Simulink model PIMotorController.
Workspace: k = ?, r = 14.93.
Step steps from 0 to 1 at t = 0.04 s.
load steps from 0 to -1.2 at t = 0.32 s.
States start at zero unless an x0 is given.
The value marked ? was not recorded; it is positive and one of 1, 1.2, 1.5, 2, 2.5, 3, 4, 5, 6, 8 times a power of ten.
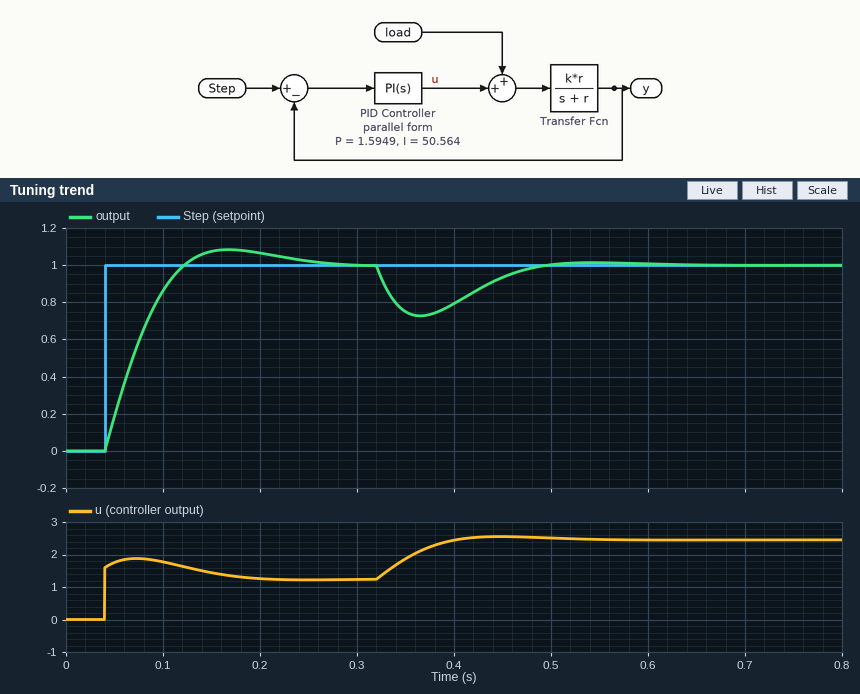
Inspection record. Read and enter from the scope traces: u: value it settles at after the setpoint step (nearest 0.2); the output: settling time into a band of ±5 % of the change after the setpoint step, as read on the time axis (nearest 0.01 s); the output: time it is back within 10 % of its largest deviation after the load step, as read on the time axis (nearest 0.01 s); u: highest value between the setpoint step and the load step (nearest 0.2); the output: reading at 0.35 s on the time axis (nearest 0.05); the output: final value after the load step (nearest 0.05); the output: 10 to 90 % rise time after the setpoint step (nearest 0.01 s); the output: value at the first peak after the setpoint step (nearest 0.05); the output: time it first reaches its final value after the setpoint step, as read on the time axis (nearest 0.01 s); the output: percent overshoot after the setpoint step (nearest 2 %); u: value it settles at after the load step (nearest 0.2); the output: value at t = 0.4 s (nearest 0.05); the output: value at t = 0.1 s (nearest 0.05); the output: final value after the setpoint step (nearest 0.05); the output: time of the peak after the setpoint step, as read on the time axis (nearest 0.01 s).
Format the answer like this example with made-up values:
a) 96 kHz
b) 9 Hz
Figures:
a) 1.2
b) 0.22 s
c) 0.47 s
d) 1.8
e) 0.75
f) 1.00
g) 0.06 s
h) 1.10
i) 0.12 s
j) 8 %
k) 2.4
l) 0.80
m) 0.85
n) 1.00
o) 0.17 s
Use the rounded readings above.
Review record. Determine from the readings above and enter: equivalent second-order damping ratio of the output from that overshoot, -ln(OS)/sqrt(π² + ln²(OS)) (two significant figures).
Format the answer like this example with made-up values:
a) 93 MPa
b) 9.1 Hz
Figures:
a) 0.63
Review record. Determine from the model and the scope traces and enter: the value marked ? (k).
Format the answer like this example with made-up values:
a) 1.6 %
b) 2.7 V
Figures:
a) 0.8
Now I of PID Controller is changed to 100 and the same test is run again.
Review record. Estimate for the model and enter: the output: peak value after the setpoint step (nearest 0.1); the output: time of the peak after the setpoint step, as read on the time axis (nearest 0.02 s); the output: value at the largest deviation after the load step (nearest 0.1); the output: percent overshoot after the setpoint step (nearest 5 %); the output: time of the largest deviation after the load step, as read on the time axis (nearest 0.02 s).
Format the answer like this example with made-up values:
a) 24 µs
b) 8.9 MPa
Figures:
a) 1.2
b) 0.12 s
c) 0.8
d) 20 %
e) 0.36 s
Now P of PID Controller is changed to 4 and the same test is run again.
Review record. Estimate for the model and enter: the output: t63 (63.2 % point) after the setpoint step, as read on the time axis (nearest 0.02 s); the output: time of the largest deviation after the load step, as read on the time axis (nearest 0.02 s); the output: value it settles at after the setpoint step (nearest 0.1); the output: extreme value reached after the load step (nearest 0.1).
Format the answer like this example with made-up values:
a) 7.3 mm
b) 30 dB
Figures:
a) 0.06 s
b) 0.36 s
c) 1.0
d) 0.8
